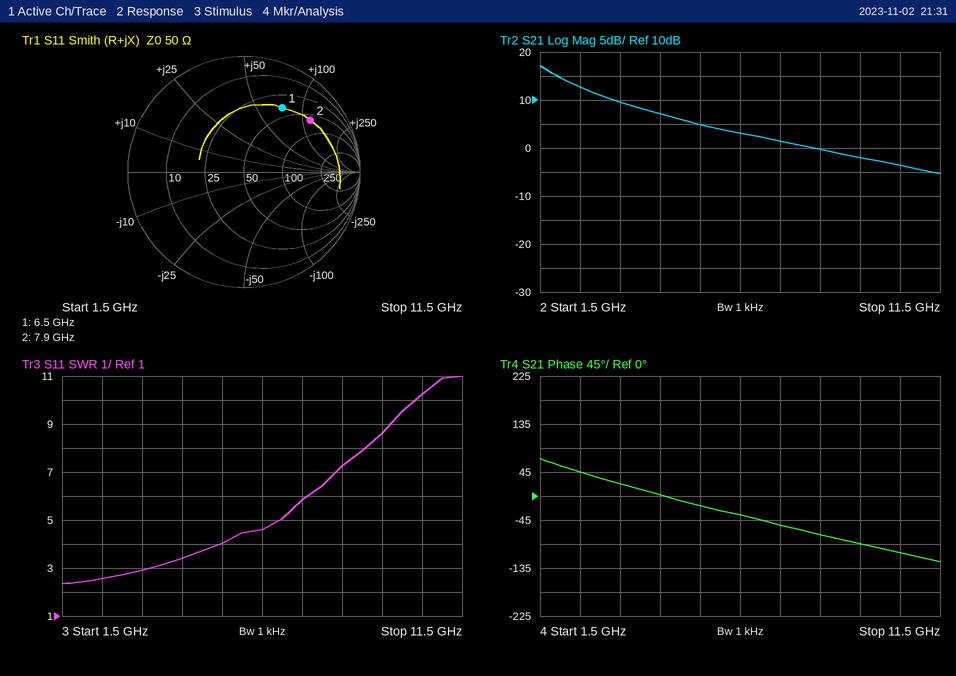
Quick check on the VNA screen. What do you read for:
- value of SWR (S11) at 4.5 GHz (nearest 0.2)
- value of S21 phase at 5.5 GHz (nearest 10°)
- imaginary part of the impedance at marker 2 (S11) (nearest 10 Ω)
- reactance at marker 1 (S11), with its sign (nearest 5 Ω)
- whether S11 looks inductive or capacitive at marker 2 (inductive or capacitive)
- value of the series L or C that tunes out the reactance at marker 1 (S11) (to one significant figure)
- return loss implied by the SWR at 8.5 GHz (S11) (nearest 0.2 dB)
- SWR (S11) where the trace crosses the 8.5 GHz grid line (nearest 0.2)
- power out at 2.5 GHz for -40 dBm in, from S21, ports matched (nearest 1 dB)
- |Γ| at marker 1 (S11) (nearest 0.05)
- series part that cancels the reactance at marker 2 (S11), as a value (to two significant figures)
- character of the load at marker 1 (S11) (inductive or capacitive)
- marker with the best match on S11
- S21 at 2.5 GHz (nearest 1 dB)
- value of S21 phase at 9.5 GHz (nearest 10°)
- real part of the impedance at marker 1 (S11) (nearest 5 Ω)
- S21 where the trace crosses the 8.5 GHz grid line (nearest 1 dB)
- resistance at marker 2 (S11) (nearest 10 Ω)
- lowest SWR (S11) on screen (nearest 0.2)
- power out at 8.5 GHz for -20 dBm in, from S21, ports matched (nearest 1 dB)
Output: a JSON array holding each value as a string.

["3.4", "-20°", "+120 Ω", "+75 Ω", "inductive", "300 fF", "2.4 dB", "7.2", "-27 dBm", "0.65", "170 fF", "inductive", "marker 1", "13 dB", "-90°", "40 Ω", "0 dB", "60 Ω", "2.4", "-20 dBm"]
